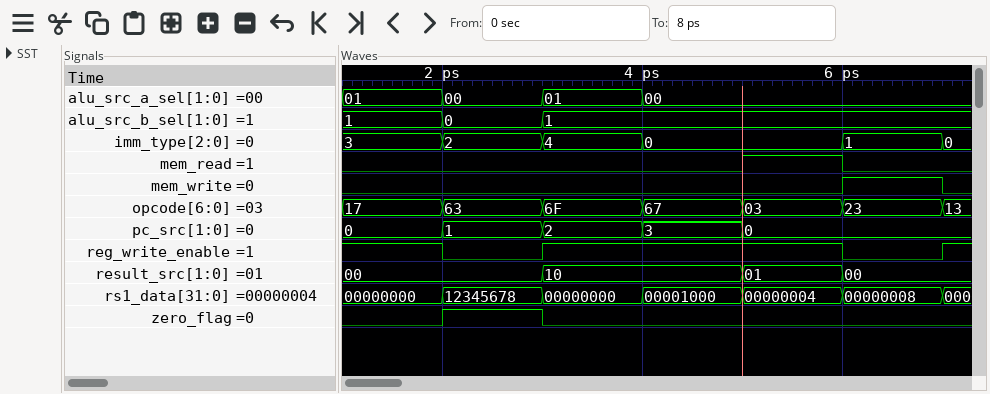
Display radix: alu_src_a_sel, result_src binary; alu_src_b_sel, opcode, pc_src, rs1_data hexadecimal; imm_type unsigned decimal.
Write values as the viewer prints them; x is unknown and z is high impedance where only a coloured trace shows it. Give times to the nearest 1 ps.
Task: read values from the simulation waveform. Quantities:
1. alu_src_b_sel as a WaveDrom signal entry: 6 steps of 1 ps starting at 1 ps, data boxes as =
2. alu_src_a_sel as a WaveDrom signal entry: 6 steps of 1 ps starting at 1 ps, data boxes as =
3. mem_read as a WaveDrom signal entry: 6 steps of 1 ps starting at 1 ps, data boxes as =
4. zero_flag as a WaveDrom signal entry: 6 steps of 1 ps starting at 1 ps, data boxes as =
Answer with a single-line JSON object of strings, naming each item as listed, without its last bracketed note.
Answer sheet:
{"alu_src_b_sel as a WaveDrom signal entry: 6 steps of 1 ps starting at 1 ps, data boxes as =": "{name: 'alu_src_b_sel', wave: '===...', data: '1 0 1'}", "alu_src_a_sel as a WaveDrom signal entry: 6 steps of 1 ps starting at 1 ps, data boxes as =": "{name: 'alu_src_a_sel', wave: '====..', data: '01 00 01 00'}", "mem_read as a WaveDrom signal entry: 6 steps of 1 ps starting at 1 ps, data boxes as =": "{name: 'mem_read', wave: '0...10'}", "zero_flag as a WaveDrom signal entry: 6 steps of 1 ps starting at 1 ps, data boxes as =": "{name: 'zero_flag', wave: '010...'}"}
